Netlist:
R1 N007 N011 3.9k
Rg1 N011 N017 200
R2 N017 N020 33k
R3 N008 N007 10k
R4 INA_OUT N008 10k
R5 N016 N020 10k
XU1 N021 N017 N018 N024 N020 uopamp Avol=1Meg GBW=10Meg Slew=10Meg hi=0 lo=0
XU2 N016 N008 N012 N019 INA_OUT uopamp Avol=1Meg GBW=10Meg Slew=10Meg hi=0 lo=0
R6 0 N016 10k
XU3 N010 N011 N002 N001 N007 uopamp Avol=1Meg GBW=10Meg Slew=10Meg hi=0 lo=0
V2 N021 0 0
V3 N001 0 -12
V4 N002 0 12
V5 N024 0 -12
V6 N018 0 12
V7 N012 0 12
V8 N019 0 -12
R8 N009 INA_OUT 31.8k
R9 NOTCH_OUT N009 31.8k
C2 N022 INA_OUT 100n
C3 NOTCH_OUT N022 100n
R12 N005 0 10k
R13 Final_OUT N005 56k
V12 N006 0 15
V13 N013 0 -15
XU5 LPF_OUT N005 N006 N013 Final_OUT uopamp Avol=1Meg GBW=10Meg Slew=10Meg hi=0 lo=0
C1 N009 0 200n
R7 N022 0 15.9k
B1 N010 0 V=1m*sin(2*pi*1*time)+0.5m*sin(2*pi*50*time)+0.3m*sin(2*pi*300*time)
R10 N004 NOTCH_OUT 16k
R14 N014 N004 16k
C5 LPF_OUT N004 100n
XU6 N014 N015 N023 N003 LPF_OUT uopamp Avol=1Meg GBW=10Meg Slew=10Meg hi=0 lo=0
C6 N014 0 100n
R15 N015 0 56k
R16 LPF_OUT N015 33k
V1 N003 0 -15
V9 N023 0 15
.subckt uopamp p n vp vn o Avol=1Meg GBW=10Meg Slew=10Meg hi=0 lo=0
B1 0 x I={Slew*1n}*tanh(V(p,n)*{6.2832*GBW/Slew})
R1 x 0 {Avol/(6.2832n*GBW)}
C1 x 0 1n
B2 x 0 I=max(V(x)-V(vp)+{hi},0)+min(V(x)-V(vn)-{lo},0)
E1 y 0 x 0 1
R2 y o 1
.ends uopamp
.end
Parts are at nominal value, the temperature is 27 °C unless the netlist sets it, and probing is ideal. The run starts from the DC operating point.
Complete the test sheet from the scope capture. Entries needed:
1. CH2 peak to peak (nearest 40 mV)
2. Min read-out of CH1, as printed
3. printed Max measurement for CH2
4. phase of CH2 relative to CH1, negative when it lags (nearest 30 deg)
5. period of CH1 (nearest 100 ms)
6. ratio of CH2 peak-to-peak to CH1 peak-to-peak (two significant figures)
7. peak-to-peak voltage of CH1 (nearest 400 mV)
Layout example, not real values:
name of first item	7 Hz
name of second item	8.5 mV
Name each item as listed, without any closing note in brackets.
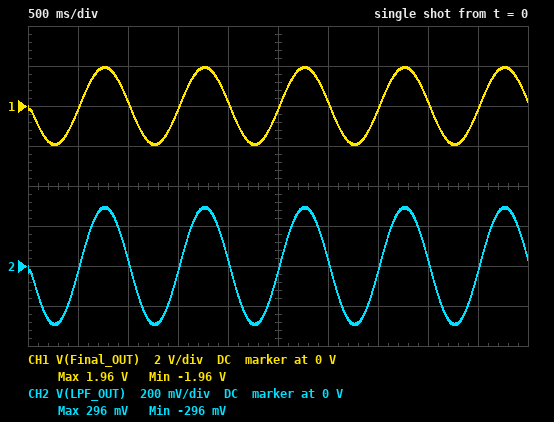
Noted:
CH2 peak to peak	600 mV
Min read-out of CH1, as printed	-1.96 V
printed Max measurement for CH2	296 mV
phase of CH2 relative to CH1, negative when it lags	0 deg
period of CH1	1.0 s
ratio of CH2 peak-to-peak to CH1 peak-to-peak	0.15
peak-to-peak voltage of CH1	4.0 V
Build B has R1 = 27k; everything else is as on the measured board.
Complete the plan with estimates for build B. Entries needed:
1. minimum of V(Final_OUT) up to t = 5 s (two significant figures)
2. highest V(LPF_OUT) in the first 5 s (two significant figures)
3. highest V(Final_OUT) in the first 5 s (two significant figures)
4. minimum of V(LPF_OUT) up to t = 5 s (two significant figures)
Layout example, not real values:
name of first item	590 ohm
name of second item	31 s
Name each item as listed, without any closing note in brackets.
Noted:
minimum of V(Final_OUT) up to t = 5 s	-3.2 V
highest V(LPF_OUT) in the first 5 s	480 mV
highest V(Final_OUT) in the first 5 s	3.2 V
minimum of V(LPF_OUT) up to t = 5 s	-480 mV
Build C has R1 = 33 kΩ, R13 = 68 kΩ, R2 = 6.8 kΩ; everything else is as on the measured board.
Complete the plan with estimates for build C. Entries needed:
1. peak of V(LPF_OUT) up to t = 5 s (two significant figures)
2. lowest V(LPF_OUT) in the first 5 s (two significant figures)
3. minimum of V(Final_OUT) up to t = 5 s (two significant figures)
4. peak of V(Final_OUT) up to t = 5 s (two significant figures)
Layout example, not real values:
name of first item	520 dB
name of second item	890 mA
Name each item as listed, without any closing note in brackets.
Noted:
peak of V(LPF_OUT) up to t = 5 s	320 mV
lowest V(LPF_OUT) in the first 5 s	-320 mV
minimum of V(Final_OUT) up to t = 5 s	-2.5 V
peak of V(Final_OUT) up to t = 5 s	2.5 V
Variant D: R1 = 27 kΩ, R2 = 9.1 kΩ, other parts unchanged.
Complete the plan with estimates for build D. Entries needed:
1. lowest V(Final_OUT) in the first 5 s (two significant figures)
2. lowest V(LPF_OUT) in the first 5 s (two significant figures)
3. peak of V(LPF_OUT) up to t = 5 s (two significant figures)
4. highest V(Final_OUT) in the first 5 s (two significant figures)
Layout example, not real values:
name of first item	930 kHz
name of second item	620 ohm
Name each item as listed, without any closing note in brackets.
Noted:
lowest V(Final_OUT) in the first 5 s	-1.9 V
lowest V(LPF_OUT) in the first 5 s	-290 mV
peak of V(LPF_OUT) up to t = 5 s	290 mV
highest V(Final_OUT) in the first 5 s	1.9 V
